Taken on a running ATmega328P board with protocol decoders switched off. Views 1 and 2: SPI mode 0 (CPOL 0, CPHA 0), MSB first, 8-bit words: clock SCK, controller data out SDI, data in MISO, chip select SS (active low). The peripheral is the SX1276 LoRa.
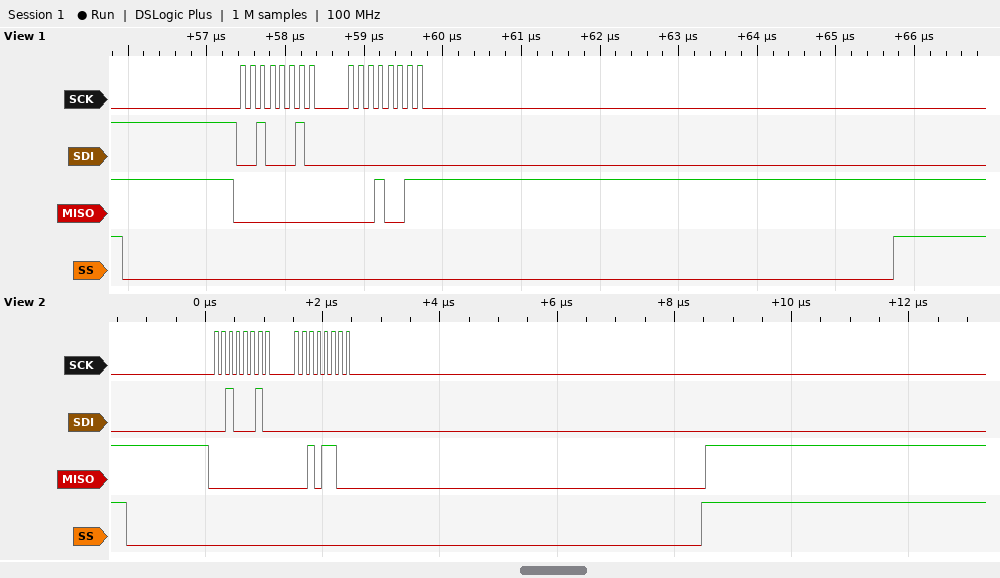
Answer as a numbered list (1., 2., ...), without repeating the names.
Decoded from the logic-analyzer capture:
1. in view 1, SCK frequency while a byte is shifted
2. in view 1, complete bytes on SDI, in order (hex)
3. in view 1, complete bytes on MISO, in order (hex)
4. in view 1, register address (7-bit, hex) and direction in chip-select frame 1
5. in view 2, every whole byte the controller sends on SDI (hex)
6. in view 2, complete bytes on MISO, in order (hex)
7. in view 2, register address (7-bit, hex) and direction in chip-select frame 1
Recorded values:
1. 8 MHz
2. 22 00
3. 00 13
4. 0x22 read
5. 22 00
6. 00 2C
7. 0x22 read
